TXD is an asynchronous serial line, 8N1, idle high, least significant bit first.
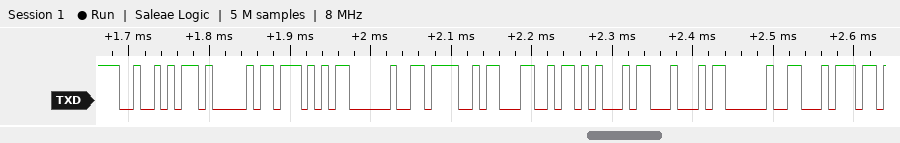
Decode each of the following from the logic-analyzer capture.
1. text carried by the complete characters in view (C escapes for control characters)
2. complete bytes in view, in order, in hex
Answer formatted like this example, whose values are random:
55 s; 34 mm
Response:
"RAW OLED t"; 0x52 0x41 0x57 0x20 0x4F 0x4C 0x45 0x44 0x20 0x74
